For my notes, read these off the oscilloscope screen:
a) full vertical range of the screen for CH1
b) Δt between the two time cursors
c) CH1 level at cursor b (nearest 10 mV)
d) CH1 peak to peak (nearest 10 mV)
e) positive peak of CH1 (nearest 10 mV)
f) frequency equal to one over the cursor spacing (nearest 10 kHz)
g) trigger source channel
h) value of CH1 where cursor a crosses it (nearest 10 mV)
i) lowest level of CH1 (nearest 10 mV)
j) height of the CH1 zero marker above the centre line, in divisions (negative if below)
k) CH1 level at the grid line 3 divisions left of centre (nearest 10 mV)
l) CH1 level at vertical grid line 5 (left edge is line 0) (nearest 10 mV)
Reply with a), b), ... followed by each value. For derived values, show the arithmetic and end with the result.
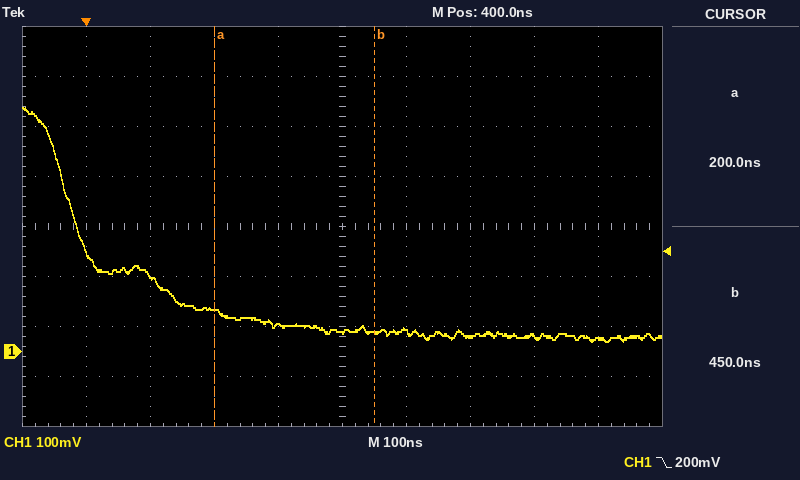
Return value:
a) 800 mV
b) 450 ns − (200 ns) = 250 ns
c) 40 mV
d) 490 mV − (20 mV) = 470 mV
e) 490 mV
f) 1 / 250 ns ≈ 4.00 MHz
g) CH1
h) 80 mV
i) 20 mV
j) -2.5 div
k) 150 mV
l) 40 mV
